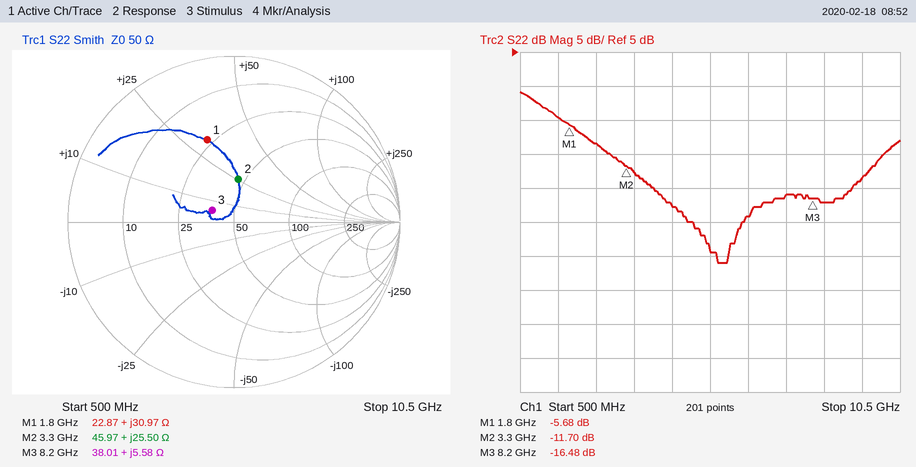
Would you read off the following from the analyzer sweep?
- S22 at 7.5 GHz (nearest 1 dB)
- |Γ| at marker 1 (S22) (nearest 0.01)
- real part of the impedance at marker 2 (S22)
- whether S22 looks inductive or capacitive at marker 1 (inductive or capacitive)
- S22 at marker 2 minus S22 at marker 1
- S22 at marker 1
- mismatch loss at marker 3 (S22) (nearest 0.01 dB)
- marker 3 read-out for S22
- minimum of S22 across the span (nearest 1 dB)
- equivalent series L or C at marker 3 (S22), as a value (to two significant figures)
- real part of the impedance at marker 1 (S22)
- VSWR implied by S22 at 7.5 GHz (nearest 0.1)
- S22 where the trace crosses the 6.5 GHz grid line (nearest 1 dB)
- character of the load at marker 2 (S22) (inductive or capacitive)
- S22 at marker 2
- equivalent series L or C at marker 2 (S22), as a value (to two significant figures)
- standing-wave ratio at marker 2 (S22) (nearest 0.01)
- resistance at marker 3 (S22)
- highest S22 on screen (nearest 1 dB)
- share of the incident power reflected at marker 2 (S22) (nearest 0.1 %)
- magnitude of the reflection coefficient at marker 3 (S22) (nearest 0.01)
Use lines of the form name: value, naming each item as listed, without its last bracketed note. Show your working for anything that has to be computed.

S22 at 7.5 GHz: -16 dB
|Γ| at marker 1 (S22): 0.52
real part of the impedance at marker 2: 45.97 Ω
whether S22 looks inductive or capacitive at marker 1: inductive
S22 at marker 2 minus S22 at marker 1: -11.7 − (-5.68) = -6.02 dB
S22 at marker 1: -5.68 dB
mismatch loss at marker 3 (S22): −10 log10(1 − 10^(-16.48/10)) ≈ 0.10 dB
marker 3 read-out for S22: -16.48 dB
minimum of S22 across the span: -26 dB
equivalent series L or C at marker 3 (S22), as a value: L = 5.58 Ω/(2π × 8.2 GHz) ≈ 108 pH, so 110 pH to two significant figures
real part of the impedance at marker 1: 22.87 Ω
VSWR implied by S22 at 7.5 GHz: |Γ| = 10^(-16/20) = 0.1585; VSWR = (1 + 0.1585)/(1 − 0.1585) ≈ 1.4
S22 where the trace crosses the 6.5 GHz grid line: -19 dB
character of the load at marker 2 (S22): inductive
S22 at marker 2: -11.70 dB
equivalent series L or C at marker 2 (S22), as a value: L = 25.5 Ω/(2π × 3.3 GHz) ≈ 1.2 nH
standing-wave ratio at marker 2 (S22): 1.70
resistance at marker 3: 38.01 Ω
highest S22 on screen: -1 dB
share of the incident power reflected at marker 2 (S22): 10^(-11.7/10) ≈ 6.8 %
magnitude of the reflection coefficient at marker 3 (S22): 0.15
